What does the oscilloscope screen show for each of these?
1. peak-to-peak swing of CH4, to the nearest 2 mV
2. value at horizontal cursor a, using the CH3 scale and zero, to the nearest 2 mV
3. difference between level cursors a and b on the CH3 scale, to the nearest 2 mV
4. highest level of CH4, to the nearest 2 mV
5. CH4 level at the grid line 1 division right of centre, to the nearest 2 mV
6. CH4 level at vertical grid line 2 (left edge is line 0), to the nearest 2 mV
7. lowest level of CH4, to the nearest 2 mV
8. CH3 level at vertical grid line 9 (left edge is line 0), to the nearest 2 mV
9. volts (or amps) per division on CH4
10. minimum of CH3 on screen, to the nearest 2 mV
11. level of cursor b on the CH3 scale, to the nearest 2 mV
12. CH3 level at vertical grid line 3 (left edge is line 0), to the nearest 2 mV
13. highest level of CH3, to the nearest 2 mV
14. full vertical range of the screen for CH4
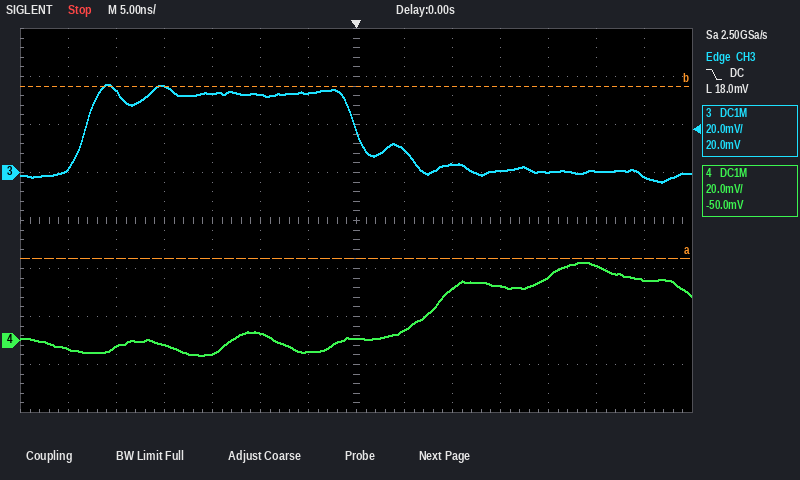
38 mV
-36 mV
72 mV
32 mV
4 mV
-2 mV
-6 mV
4 mV
20 mV
-4 mV
36 mV
36 mV
36 mV
160 mV
